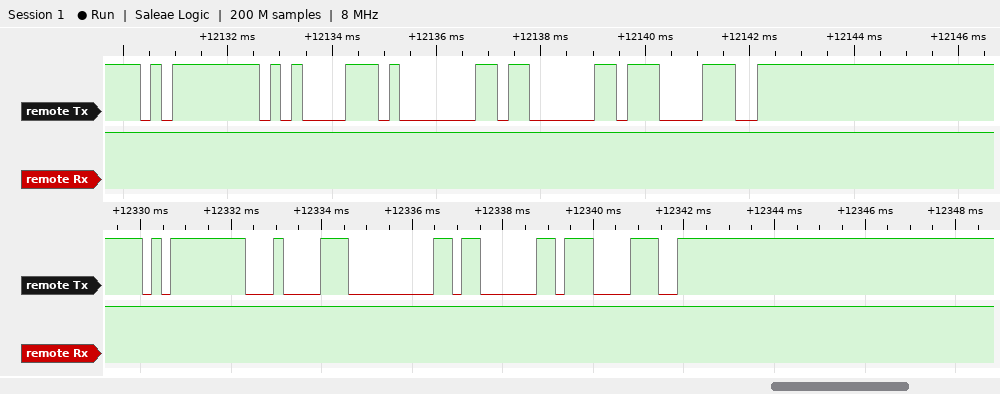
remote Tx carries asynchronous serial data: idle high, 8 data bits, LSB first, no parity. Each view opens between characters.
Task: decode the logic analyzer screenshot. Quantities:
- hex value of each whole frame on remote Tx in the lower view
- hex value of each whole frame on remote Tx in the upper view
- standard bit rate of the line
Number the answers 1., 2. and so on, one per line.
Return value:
1. FD, 84, 00, 03, 87, FE
2. FD, 85, 01, 03, 87, FE
3. 4800 baud
